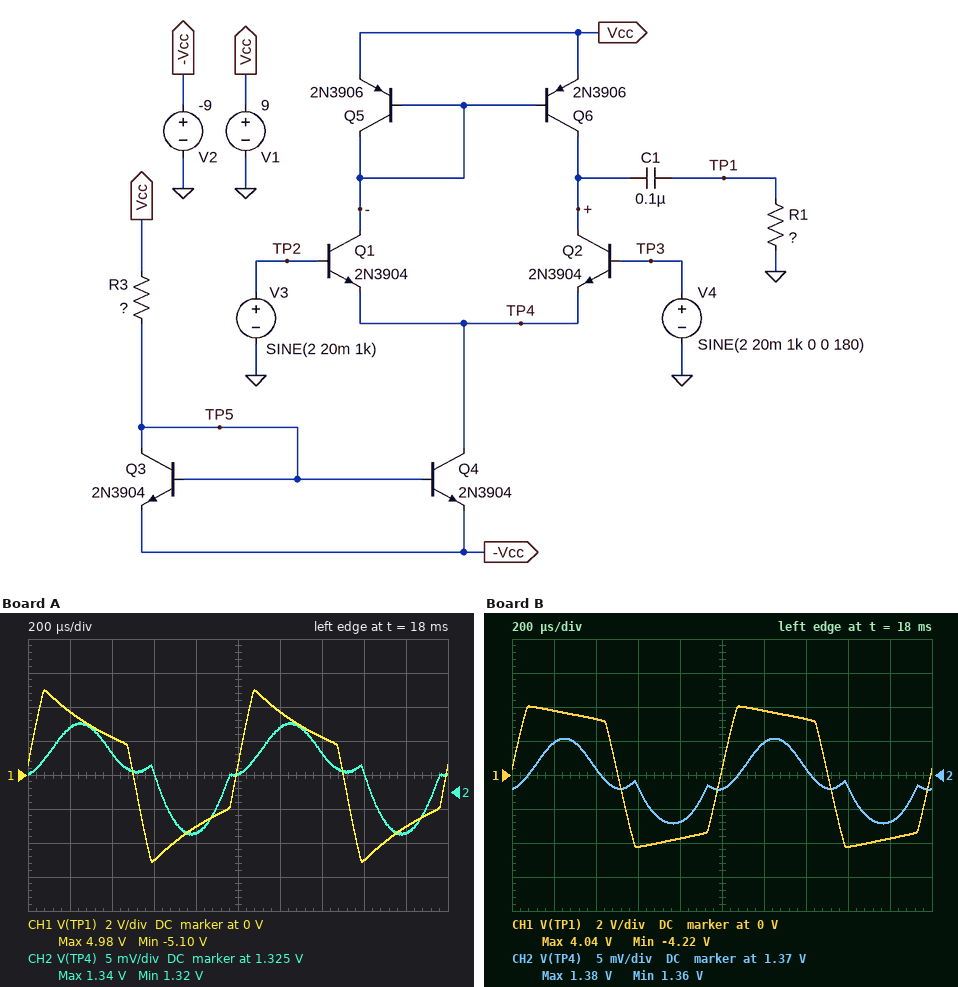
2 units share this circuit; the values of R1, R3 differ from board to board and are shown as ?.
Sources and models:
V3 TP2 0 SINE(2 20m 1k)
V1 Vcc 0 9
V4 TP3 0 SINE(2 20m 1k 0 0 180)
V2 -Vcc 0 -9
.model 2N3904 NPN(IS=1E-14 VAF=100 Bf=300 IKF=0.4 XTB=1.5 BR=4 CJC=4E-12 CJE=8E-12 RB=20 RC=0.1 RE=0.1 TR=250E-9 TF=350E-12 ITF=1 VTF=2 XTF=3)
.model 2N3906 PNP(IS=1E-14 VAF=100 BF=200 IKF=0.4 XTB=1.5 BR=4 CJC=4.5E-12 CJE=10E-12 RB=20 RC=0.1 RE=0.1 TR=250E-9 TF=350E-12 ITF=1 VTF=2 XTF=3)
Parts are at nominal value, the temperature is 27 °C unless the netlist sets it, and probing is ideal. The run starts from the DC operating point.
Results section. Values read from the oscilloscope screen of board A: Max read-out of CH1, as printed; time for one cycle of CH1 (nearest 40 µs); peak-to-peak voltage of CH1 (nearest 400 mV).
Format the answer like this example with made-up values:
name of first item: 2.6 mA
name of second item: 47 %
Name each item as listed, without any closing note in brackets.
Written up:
Max read-out of CH1, as printed: 4.98 V
time for one cycle of CH1: 1.00 ms
peak-to-peak voltage of CH1: 10.0 V
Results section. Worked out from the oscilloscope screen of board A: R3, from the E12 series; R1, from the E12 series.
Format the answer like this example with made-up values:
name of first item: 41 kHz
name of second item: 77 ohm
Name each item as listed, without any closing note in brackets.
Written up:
R3, from the E12 series: 4.7 kΩ
R1, from the E12 series: 3.9 kΩ
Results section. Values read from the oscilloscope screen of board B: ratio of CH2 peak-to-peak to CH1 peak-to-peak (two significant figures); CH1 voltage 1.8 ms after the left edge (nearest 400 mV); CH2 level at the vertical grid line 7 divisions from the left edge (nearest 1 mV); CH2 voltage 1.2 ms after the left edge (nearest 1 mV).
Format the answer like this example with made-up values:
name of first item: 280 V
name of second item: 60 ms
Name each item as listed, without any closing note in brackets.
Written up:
ratio of CH2 peak-to-peak to CH1 peak-to-peak: 0.0015
CH1 voltage 1.8 ms after the left edge: -3.6 V
CH2 level at the vertical grid line 7 divisions from the left edge: 1.371 V
CH2 voltage 1.2 ms after the left edge: 1.375 V
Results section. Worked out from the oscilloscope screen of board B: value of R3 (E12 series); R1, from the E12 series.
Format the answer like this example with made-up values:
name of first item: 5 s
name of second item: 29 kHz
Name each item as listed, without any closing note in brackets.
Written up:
value of R3: 22 kΩ
R1, from the E12 series: 15 kΩ
